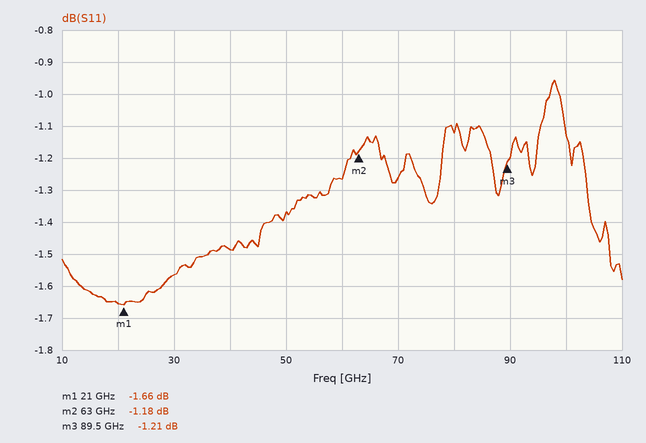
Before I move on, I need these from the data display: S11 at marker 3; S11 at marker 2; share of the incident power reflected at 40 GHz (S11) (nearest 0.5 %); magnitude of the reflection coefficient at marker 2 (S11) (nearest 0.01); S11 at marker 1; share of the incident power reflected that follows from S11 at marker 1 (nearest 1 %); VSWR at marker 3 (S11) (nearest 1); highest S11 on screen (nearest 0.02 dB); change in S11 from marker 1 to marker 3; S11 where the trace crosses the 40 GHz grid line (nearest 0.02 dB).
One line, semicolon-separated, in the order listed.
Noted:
-1.21 dB; -1.18 dB; 71.0 %; 0.87; -1.66 dB; 68 %; 14; -0.96 dB; 0.45 dB; -1.48 dB
